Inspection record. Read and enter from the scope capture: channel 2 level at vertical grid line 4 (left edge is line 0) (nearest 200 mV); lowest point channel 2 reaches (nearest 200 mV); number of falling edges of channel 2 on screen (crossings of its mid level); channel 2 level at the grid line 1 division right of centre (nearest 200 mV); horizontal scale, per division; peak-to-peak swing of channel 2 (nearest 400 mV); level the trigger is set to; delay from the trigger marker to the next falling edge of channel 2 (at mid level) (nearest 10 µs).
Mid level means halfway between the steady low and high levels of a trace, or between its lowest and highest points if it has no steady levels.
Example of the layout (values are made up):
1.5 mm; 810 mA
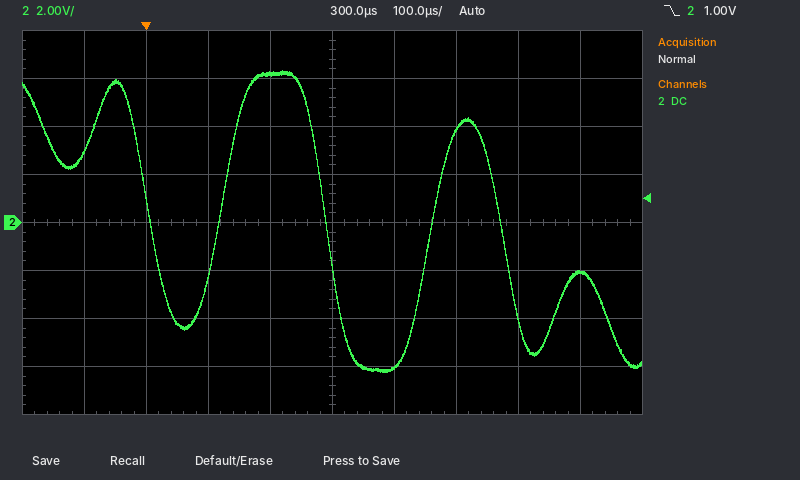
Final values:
6.2 V; -6.2 V; 3; -6.0 V; 100 µs; 12.4 V; 1.00 V; 10 µs
